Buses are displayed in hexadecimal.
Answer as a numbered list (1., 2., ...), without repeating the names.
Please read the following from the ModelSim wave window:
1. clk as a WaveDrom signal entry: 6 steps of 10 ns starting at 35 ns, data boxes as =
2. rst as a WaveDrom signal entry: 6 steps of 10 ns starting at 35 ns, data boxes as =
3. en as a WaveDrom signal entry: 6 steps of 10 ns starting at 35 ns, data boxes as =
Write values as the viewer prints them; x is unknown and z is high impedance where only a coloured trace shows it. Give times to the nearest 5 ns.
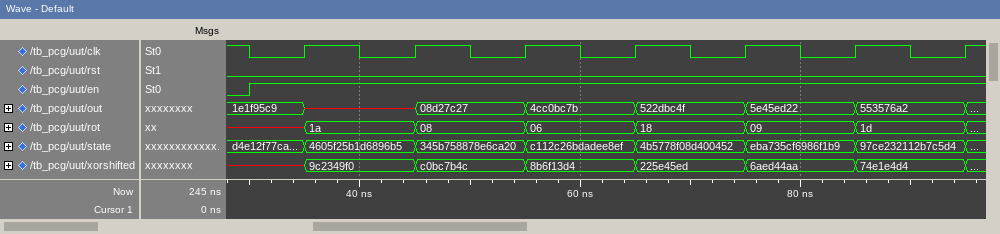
1. {name: 'clk', wave: 'p.....'}
2. {name: 'rst', wave: '0.....'}
3. {name: 'en', wave: '1.....'}
